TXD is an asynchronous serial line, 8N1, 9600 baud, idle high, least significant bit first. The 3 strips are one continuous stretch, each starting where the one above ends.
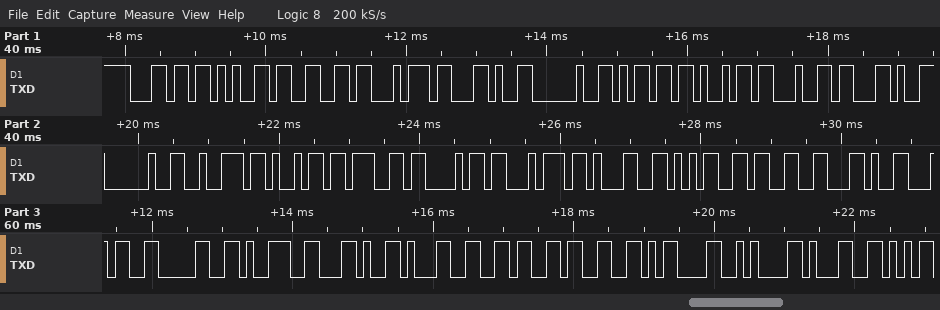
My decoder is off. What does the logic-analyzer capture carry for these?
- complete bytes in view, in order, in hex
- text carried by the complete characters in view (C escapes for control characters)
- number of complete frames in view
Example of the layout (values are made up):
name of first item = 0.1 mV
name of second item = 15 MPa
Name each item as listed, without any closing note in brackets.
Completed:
complete bytes in view, in order, in hex = 6C 65 66 74 2C 20 6D 69 64 2C 20 72 69 67 68 74 31 35 33 2C 34 30 39 2C 31 36 33 0D 0A 31
text carried by the complete characters in view = "left, mid, right153,409,163\r\n1"
number of complete frames in view = 30
